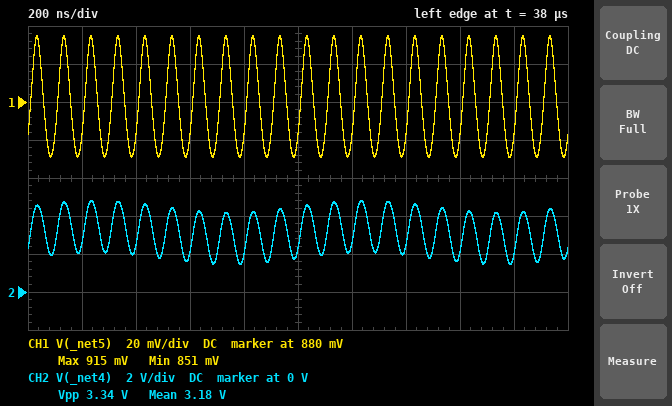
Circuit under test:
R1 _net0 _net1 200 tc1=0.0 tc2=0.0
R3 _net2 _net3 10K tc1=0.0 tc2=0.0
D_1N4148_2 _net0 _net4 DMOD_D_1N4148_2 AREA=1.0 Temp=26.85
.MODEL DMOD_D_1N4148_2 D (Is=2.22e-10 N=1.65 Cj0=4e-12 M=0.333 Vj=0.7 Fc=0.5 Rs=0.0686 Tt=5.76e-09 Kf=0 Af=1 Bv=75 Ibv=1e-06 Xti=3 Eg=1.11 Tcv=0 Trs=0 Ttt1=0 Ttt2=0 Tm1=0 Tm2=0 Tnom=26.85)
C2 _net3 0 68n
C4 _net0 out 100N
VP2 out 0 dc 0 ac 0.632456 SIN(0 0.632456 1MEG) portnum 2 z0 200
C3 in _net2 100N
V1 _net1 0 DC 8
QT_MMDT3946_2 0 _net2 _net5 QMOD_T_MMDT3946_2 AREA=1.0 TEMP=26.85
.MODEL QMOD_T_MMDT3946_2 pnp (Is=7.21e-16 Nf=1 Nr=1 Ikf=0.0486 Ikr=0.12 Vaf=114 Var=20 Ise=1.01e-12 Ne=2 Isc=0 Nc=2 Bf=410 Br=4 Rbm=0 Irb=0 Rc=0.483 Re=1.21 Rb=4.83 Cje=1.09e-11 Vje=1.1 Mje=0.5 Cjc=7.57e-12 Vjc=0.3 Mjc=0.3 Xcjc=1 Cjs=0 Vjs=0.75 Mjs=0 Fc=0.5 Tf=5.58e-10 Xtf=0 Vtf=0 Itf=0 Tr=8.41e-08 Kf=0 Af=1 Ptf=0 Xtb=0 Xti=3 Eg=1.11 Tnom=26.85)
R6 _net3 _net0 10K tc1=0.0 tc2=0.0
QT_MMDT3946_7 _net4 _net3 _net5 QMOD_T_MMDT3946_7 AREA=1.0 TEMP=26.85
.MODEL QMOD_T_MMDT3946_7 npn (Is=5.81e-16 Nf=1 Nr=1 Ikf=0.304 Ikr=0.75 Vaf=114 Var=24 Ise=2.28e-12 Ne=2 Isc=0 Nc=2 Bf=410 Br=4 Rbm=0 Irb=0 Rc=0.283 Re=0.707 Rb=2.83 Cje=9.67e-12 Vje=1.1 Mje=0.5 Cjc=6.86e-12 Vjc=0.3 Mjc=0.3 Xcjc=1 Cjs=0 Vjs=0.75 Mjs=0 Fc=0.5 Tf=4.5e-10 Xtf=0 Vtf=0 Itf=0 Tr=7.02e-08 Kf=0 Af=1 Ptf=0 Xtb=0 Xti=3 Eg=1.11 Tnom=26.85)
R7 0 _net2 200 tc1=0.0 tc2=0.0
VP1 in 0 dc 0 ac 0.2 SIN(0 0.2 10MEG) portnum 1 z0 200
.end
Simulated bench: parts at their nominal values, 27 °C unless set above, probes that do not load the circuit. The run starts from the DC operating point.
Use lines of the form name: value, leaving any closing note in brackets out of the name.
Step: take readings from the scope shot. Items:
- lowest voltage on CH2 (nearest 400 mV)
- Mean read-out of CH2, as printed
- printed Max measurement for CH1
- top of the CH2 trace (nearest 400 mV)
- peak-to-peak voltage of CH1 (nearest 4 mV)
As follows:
lowest voltage on CH2: 1.6 V
Mean read-out of CH2, as printed: 3.18 V
printed Max measurement for CH1: 915 mV
top of the CH2 trace: 4.8 V
peak-to-peak voltage of CH1: 64 mV
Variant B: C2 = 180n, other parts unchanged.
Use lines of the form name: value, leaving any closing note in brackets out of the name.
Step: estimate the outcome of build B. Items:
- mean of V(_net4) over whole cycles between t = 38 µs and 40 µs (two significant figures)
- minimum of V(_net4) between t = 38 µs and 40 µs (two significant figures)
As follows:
mean of V(_net4) over whole cycles between t = 38 µs and 40 µs: 3.1 V
minimum of V(_net4) between t = 38 µs and 40 µs: 1.4 V
